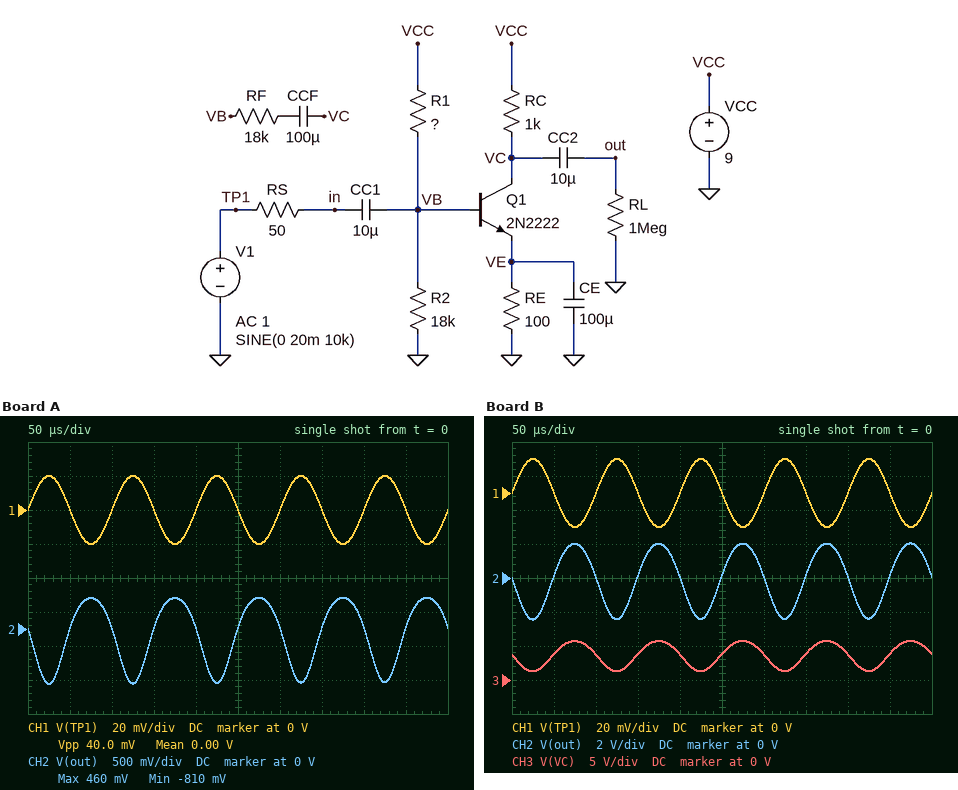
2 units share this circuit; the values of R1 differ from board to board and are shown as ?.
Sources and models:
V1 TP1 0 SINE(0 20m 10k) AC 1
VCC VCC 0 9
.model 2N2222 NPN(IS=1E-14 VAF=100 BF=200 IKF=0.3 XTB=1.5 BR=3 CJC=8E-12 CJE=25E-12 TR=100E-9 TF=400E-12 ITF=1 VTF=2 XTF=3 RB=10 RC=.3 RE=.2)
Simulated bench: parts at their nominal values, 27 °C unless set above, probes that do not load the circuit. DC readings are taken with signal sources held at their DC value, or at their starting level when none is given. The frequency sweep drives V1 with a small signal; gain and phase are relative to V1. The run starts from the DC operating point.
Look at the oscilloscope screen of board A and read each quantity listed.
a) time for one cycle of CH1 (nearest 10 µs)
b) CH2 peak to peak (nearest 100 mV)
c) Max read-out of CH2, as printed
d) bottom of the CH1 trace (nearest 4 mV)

100 µs
1.3 V
460 mV
-20 mV
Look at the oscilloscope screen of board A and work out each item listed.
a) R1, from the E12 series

180 kΩ
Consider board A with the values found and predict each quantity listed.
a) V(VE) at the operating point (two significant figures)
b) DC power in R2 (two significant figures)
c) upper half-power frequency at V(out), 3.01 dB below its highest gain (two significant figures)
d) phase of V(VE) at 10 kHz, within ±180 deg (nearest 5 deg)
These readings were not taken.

94 mV
31 µW
13 MHz
-90 deg
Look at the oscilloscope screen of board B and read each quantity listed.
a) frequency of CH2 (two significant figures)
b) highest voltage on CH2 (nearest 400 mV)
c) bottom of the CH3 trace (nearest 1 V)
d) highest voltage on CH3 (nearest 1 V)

10 kHz
2.0 V
1 V
6 V
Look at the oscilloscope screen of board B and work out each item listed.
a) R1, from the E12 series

82 kΩ
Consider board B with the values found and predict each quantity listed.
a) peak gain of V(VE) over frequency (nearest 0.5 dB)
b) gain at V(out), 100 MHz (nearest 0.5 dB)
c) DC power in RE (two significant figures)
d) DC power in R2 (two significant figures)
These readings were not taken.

-4.5 dB
12.5 dB
2.8 mW
84 µW
